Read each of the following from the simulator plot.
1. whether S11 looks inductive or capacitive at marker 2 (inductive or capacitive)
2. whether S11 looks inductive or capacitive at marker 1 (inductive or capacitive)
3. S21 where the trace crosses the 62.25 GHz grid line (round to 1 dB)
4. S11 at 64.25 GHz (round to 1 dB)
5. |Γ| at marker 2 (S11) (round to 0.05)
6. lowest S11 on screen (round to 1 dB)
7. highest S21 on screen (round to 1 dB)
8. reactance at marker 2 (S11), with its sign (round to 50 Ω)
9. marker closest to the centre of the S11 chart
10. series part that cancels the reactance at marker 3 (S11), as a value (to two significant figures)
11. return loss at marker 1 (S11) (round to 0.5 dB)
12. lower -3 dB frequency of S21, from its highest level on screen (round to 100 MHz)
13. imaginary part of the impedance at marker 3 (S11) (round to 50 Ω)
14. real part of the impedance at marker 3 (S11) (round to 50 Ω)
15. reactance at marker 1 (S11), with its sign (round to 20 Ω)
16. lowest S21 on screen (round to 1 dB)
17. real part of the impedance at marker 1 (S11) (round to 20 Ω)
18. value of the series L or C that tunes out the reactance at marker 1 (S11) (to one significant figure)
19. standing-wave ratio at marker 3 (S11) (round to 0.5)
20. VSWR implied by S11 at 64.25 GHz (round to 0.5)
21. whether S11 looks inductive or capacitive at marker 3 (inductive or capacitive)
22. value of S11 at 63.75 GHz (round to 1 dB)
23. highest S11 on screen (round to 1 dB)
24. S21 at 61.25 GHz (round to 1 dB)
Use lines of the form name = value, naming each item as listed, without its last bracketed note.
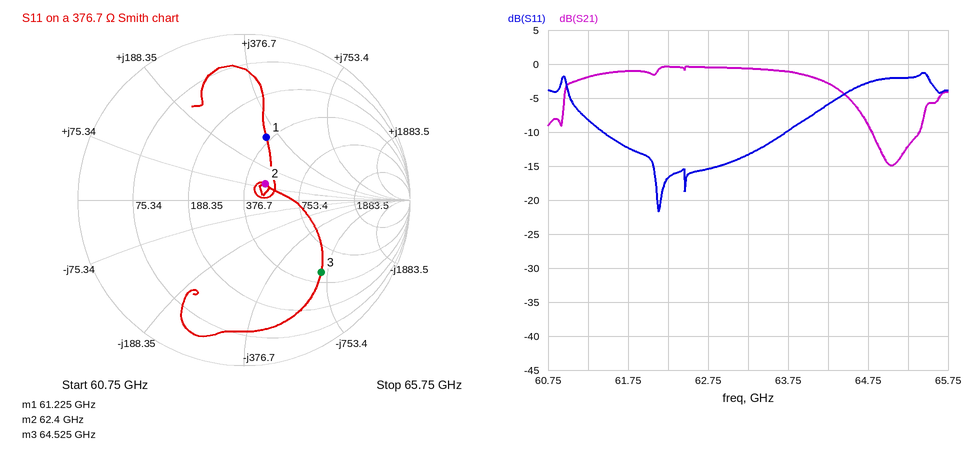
whether S11 looks inductive or capacitive at marker 2 = inductive
whether S11 looks inductive or capacitive at marker 1 = inductive
S21 where the trace crosses the 62.25 GHz grid line = 0 dB
S11 at 64.25 GHz = -6 dB
|Γ| at marker 2 (S11) = 0.15
lowest S11 on screen = -22 dB
highest S21 on screen = 0 dB
reactance at marker 2 (S11), with its sign = +100 Ω
marker closest to the centre of the S11 chart = marker 2
series part that cancels the reactance at marker 3 (S11), as a value = 1.7 nH
return loss at marker 1 (S11) = 8.0 dB
lower -3 dB frequency of S21, from its highest level on screen = 61.0 GHz
imaginary part of the impedance at marker 3 (S11) = -700 Ω
real part of the impedance at marker 3 (S11) = 450 Ω
reactance at marker 1 (S11), with its sign = +320 Ω
lowest S21 on screen = -15 dB
real part of the impedance at marker 1 (S11) = 360 Ω
value of the series L or C that tunes out the reactance at marker 1 (S11) = 8 fF
standing-wave ratio at marker 3 (S11) = 4.5
VSWR implied by S11 at 64.25 GHz = 3.0
whether S11 looks inductive or capacitive at marker 3 = capacitive
value of S11 at 63.75 GHz = -10 dB
highest S11 on screen = -1 dB
S21 at 61.25 GHz = -2 dB
